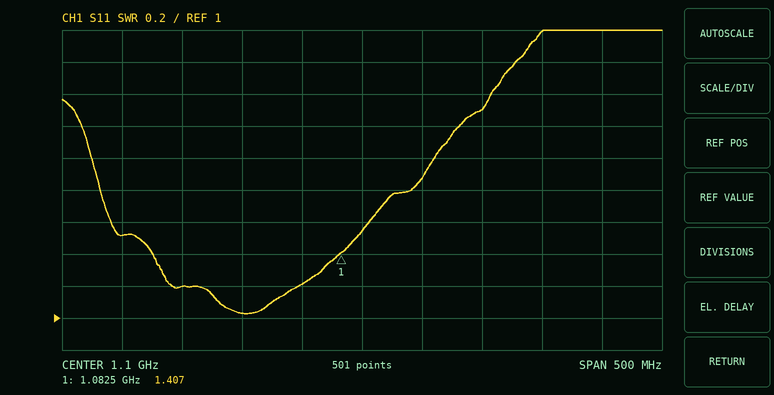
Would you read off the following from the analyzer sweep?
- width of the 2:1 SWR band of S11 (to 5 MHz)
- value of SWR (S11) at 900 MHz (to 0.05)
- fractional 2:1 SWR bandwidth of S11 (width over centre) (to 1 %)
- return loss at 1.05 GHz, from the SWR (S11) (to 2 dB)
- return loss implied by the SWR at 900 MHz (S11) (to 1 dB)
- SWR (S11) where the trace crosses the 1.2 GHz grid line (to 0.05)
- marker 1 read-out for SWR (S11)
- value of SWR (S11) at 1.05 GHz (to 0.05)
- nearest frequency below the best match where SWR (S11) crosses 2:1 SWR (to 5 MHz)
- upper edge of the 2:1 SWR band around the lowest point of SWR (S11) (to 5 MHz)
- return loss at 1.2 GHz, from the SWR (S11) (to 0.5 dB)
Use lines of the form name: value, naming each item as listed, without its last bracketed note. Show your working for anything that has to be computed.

width of the 2:1 SWR band of S11: 1.160 GHz − 875 MHz = 285 MHz
value of SWR (S11) at 900 MHz: 1.50
fractional 2:1 SWR bandwidth of S11 (width over centre): 285 MHz / 1.0175 GHz ≈ 28 %
return loss at 1.05 GHz, from the SWR (S11): −20 log10((1.2 − 1)/(1.2 + 1)) ≈ 20.8 dB, so 20 dB to the nearest 2 dB
return loss implied by the SWR at 900 MHz (S11): −20 log10((1.5 − 1)/(1.5 + 1)) ≈ 14 dB
SWR (S11) where the trace crosses the 1.2 GHz grid line: 2.30
marker 1 read-out for SWR: 1.407
value of SWR (S11) at 1.05 GHz: 1.20
nearest frequency below the best match where SWR (S11) crosses 2:1 SWR: 875 MHz
upper edge of the 2:1 SWR band around the lowest point of SWR (S11): 1.160 GHz
return loss at 1.2 GHz, from the SWR (S11): −20 log10((2.3 − 1)/(2.3 + 1)) ≈ 8.09 dB, so 8.0 dB to the nearest 0.5 dB
